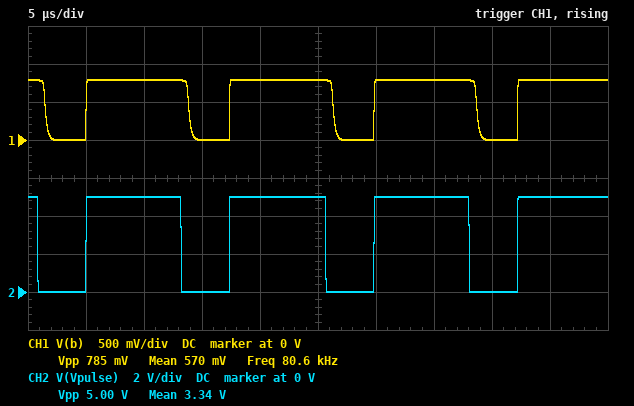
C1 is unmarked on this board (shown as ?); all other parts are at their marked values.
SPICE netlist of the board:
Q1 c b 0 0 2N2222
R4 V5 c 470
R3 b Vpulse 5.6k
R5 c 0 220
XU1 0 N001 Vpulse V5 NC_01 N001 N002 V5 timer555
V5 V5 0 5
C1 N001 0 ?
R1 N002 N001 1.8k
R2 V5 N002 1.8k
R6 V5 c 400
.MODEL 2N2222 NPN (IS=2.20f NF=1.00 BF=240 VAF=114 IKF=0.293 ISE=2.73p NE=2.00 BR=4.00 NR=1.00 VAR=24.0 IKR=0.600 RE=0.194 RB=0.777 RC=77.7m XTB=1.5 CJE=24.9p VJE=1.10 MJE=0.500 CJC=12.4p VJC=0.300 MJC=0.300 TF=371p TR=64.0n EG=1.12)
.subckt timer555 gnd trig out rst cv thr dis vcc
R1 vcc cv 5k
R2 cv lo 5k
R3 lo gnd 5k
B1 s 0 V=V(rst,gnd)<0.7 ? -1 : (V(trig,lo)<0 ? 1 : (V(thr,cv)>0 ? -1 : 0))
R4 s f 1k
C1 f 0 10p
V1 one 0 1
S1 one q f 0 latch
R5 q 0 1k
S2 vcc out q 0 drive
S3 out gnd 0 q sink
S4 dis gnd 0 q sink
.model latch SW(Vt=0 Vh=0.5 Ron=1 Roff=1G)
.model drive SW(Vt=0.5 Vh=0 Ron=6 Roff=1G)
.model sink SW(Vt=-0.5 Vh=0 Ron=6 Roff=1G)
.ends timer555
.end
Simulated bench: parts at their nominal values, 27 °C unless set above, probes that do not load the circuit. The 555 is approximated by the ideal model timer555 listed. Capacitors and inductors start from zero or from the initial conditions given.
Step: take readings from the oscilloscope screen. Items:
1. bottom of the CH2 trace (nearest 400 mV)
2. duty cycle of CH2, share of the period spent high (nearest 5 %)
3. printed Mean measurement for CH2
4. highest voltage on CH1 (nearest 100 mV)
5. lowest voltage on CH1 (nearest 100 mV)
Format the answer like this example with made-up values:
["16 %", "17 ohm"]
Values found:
["0 V", "65 %", "3.34 V", "800 mV", "0 V"]
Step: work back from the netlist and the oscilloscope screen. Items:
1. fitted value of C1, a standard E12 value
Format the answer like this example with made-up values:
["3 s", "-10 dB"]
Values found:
["3.3 nF"]
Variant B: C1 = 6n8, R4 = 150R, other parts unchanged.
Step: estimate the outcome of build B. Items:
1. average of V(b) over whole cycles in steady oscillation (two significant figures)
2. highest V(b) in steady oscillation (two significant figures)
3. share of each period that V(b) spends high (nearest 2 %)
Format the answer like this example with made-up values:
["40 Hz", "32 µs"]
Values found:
["560 mV", "810 mV", "68 %"]
